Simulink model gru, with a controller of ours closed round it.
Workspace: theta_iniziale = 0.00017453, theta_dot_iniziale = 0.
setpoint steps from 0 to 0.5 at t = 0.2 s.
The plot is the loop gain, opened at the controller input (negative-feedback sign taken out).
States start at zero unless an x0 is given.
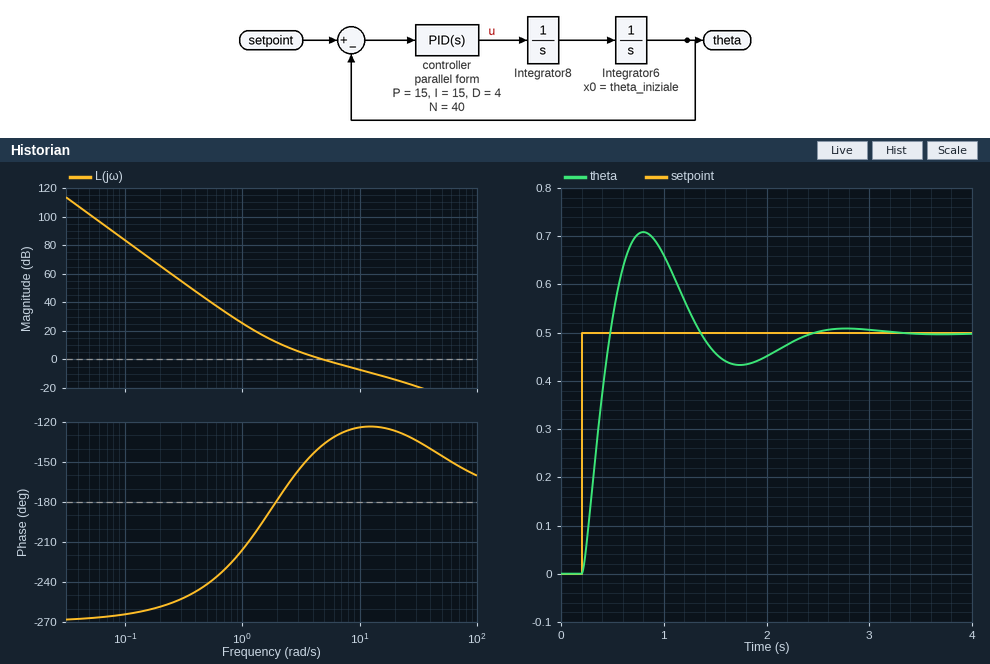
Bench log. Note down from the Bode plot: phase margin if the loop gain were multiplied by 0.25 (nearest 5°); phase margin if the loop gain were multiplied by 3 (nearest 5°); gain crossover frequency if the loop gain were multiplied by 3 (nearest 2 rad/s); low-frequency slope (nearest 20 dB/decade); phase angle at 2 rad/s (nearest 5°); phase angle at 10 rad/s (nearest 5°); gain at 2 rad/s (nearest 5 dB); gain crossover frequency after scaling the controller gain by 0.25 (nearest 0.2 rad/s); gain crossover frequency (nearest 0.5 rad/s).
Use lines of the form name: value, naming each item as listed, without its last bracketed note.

phase margin if the loop gain were multiplied by 0.25: 0°
phase margin if the loop gain were multiplied by 3: 55°
gain crossover frequency if the loop gain were multiplied by 3: 12 rad/s
low-frequency slope: -60 dB/decade
phase angle at 2 rad/s: -180°
phase angle at 10 rad/s: -125°
gain at 2 rad/s: 10 dB
gain crossover frequency after scaling the controller gain by 0.25: 2.0 rad/s
gain crossover frequency: 5.0 rad/s
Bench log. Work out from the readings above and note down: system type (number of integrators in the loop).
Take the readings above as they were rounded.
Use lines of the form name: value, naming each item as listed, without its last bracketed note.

system type: 3
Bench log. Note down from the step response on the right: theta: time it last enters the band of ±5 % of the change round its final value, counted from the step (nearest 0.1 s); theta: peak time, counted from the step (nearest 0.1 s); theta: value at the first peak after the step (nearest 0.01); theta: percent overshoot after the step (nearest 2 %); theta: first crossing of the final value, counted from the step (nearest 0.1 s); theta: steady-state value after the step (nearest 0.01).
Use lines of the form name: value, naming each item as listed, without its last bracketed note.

theta: time it last enters the band of ±5 % of the change round its final value, counted from the step: 2.0 s
theta: peak time, counted from the step: 0.6 s
theta: value at the first peak after the step: 0.71
theta: percent overshoot after the step: 42 %
theta: first crossing of the final value, counted from the step: 0.3 s
theta: steady-state value after the step: 0.50
